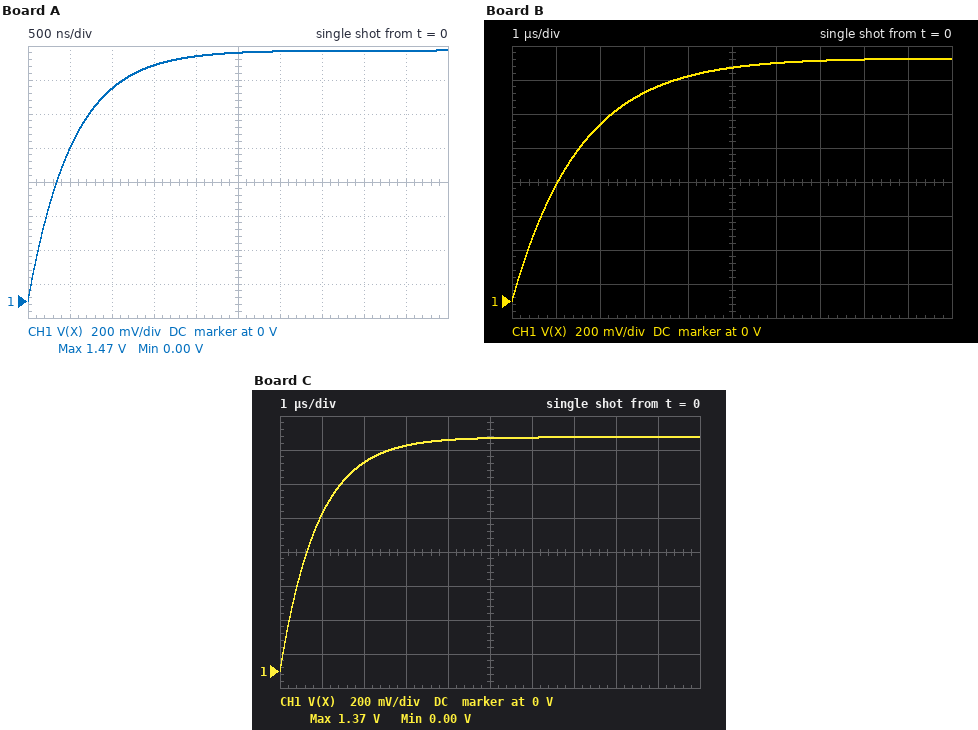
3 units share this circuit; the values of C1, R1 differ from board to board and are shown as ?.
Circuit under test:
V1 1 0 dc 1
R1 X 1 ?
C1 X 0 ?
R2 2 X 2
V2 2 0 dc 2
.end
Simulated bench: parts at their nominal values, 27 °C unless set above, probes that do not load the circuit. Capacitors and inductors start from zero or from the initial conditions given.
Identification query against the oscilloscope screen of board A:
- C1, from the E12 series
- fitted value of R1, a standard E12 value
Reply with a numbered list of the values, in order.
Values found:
1. 560 nF
2. 1.8 Ω
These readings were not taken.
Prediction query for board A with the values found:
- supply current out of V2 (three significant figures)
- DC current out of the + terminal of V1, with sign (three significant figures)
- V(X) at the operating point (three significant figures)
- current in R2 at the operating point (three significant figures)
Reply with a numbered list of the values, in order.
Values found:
1. 263 mA
2. -263 mA
3. 1.47 V
4. 263 mA
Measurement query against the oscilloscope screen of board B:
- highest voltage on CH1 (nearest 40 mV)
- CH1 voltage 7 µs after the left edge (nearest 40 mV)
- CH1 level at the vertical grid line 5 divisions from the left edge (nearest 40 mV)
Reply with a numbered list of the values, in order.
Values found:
1. 1.44 V
2. 1.40 V
3. 1.36 V
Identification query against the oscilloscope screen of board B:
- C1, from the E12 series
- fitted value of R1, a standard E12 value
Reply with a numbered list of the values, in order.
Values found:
1. 1.8 µF
2. 1.5 Ω
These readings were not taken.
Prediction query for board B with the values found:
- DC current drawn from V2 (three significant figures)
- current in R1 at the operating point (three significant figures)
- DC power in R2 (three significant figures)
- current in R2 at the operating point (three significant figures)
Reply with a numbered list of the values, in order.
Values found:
1. 286 mA
2. 286 mA
3. 163 mW
4. 286 mA
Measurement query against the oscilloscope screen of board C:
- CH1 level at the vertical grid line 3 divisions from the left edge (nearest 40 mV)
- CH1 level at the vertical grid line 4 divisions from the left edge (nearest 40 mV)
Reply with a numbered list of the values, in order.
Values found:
1. 1.32 V
2. 1.36 V
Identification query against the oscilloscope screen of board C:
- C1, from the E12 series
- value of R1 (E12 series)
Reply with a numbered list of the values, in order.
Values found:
1. 1.2 µF
2. 1.2 Ω
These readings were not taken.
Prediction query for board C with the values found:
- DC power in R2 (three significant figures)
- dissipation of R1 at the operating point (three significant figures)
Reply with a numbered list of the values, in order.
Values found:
1. 195 mW
2. 117 mW
